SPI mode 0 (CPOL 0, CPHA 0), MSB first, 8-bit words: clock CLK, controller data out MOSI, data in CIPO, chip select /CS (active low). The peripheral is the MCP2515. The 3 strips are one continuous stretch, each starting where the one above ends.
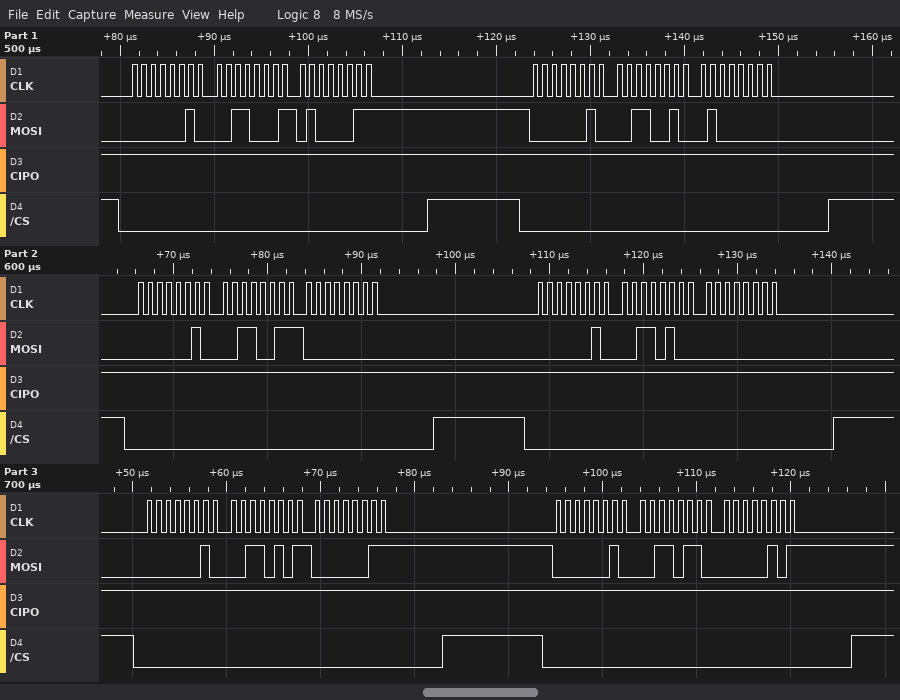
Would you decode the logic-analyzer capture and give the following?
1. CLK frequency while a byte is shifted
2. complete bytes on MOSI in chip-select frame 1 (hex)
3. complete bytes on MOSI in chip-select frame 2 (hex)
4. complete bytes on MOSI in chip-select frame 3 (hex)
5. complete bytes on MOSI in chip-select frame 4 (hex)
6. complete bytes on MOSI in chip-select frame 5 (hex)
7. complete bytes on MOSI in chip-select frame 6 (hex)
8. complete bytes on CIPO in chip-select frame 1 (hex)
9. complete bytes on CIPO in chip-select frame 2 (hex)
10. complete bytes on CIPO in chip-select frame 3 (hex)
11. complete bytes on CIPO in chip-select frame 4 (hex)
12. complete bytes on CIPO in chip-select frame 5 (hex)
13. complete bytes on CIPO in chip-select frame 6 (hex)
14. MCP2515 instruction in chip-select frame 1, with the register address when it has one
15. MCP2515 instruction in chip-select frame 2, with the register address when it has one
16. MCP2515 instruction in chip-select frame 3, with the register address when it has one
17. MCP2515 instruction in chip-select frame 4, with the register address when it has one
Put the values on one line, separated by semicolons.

1 MHz; 02 31 43; 02 32 40; 02 33 00; 02 34 00; 02 35 03; 02 36 05; FF FF FF; FF FF FF; FF FF FF; FF FF FF; FF FF FF; FF FF FF; WRITE 0x31; WRITE 0x32; WRITE 0x33; WRITE 0x34
